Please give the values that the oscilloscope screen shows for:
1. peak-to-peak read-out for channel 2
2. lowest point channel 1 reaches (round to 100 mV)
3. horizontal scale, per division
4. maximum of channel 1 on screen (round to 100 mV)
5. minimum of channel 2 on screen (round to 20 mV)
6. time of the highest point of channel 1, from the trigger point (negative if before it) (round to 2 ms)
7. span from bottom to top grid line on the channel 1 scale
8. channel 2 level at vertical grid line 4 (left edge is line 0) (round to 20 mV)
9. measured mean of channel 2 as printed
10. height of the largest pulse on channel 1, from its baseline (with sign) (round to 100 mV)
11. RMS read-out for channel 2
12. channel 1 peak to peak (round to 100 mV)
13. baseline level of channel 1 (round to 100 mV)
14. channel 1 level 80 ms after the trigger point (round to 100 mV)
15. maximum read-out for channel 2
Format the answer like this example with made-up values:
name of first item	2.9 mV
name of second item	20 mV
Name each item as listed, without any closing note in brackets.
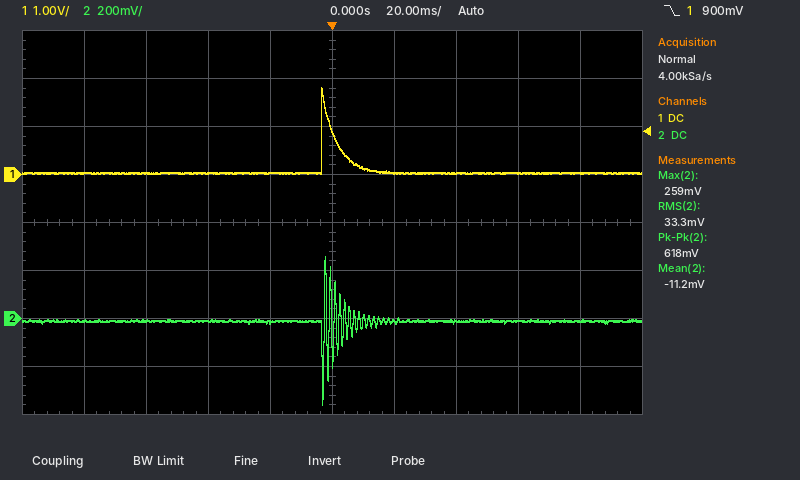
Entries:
peak-to-peak read-out for channel 2	618 mV
lowest point channel 1 reaches	0.0 V
horizontal scale, per division	20 ms
maximum of channel 1 on screen	1.8 V
minimum of channel 2 on screen	-360 mV
time of the highest point of channel 1, from the trigger point (negative if before it)	-4 ms
span from bottom to top grid line on the channel 1 scale	8 V
channel 2 level at vertical grid line 4 (left edge is line 0)	-20 mV
measured mean of channel 2 as printed	-11.2 mV
height of the largest pulse on channel 1, from its baseline (with sign)	+1.8 V
RMS read-out for channel 2	33.3 mV
channel 1 peak to peak	1.8 V
baseline level of channel 1	0.0 V
channel 1 level 80 ms after the trigger point	0.0 V
maximum read-out for channel 2	259 mV
